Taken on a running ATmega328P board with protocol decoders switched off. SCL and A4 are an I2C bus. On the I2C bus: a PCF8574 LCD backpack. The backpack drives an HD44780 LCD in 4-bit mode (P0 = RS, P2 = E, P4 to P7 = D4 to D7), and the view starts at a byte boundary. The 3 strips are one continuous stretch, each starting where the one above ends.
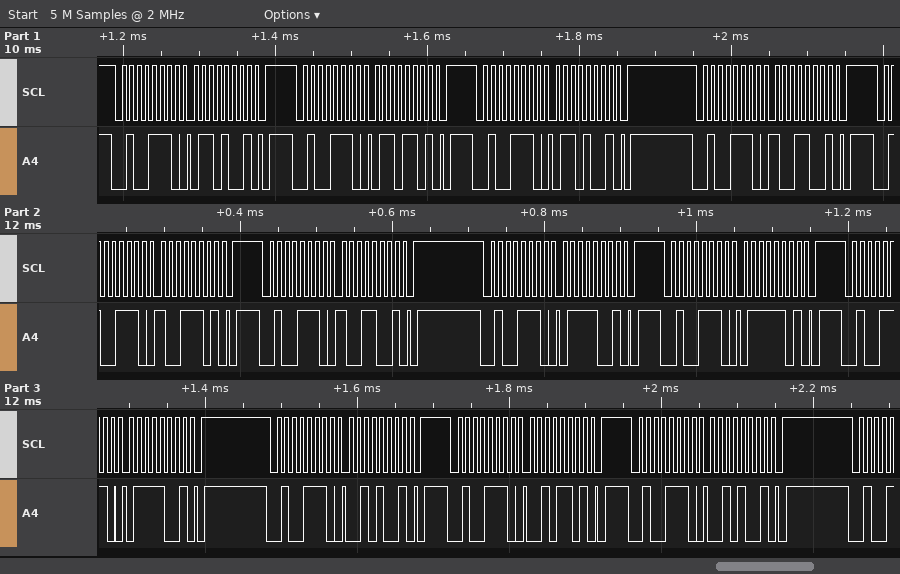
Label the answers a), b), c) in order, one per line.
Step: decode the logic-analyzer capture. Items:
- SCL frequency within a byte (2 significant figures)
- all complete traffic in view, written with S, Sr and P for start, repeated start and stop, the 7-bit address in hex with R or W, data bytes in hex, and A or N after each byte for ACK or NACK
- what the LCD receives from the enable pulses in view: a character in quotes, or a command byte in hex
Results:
a) 100 kHz
b) S 27W A 69 A P S 27W A 6D A P S 27W A 69 A P S 27W A 99 A P S 27W A 9D A P S 27W A 99 A P S 27W A 79 A P S 27W A 7D A P S 27W A 79 A P S 27W A 29 A P S 27W A 2D A P S 27W A 29 A P
c) 'i' 'r'
